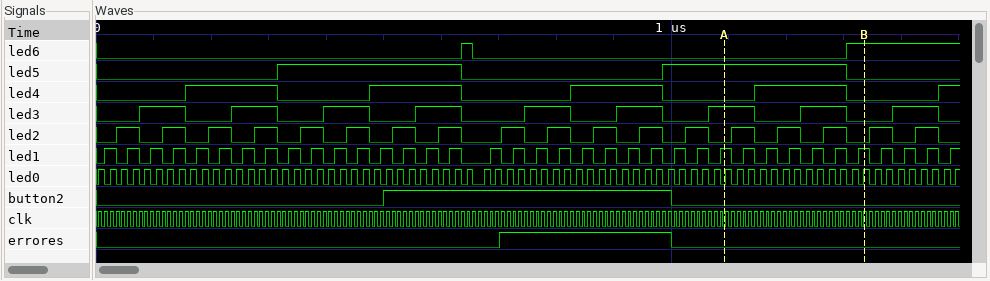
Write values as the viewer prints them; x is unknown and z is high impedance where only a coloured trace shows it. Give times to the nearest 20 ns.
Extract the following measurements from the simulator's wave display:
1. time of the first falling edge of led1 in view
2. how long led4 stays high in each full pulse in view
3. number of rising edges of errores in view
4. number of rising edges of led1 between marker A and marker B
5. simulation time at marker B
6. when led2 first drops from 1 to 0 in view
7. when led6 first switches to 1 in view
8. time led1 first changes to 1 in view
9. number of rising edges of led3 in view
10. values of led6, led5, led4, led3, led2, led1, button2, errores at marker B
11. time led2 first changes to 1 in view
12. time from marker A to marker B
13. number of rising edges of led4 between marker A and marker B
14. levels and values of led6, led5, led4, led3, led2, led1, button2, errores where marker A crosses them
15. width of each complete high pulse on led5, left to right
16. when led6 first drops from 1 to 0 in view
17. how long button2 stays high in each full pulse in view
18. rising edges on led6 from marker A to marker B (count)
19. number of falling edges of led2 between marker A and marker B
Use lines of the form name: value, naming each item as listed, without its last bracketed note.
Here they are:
time of the first falling edge of led1 in view: 40 ns
how long led4 stays high in each full pulse in view: 160 ns, 160 ns, 160 ns, 160 ns
number of rising edges of errores in view: 1
number of rising edges of led1 between marker A and marker B: 6
simulation time at marker B: 1340 ns
when led2 first drops from 1 to 0 in view: 80 ns
when led6 first switches to 1 in view: 640 ns
time led1 first changes to 1 in view: 20 ns
number of rising edges of led3 in view: 9
values of led6, led5, led4, led3, led2, led1, button2, errores at marker B: led6=1, led5=0, led4=0, led3=0, led2=0, led1=1, button2=0, errores=0
time led2 first changes to 1 in view: 40 ns
time from marker A to marker B: 240 ns
number of rising edges of led4 between marker A and marker B: 1
levels and values of led6, led5, led4, led3, led2, led1, button2, errores where marker A crosses them: led6=0, led5=1, led4=0, led3=1, led2=0, led1=1, button2=0, errores=0
width of each complete high pulse on led5, left to right: 320 ns, 320 ns
when led6 first drops from 1 to 0 in view: 660 ns
how long button2 stays high in each full pulse in view: 500 ns
rising edges on led6 from marker A to marker B: 1
number of falling edges of led2 between marker A and marker B: 3
